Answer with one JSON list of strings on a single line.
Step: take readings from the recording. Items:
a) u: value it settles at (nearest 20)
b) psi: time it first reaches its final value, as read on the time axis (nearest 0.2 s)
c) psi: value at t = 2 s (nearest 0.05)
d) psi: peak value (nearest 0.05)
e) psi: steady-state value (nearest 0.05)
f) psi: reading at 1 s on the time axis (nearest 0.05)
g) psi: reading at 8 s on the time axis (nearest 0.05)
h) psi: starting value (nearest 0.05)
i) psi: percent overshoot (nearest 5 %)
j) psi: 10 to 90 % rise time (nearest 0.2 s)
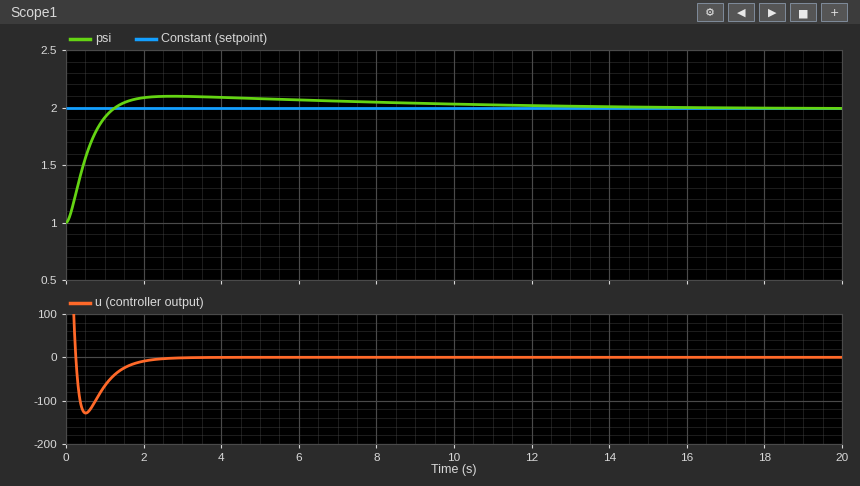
["0", "1.2 s", "2.10", "2.10", "2.00", "1.90", "2.05", "1.00", "10 %", "0.8 s"]
